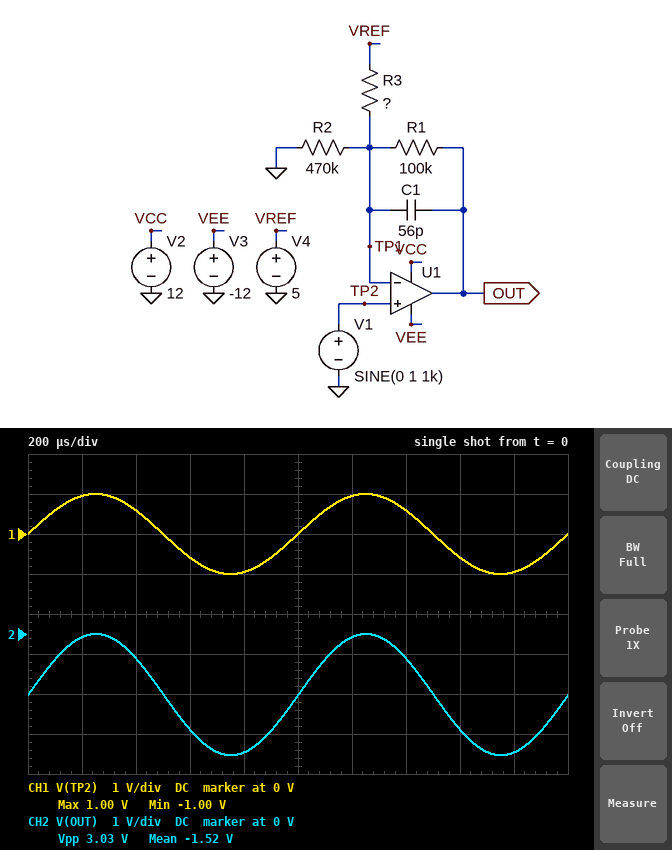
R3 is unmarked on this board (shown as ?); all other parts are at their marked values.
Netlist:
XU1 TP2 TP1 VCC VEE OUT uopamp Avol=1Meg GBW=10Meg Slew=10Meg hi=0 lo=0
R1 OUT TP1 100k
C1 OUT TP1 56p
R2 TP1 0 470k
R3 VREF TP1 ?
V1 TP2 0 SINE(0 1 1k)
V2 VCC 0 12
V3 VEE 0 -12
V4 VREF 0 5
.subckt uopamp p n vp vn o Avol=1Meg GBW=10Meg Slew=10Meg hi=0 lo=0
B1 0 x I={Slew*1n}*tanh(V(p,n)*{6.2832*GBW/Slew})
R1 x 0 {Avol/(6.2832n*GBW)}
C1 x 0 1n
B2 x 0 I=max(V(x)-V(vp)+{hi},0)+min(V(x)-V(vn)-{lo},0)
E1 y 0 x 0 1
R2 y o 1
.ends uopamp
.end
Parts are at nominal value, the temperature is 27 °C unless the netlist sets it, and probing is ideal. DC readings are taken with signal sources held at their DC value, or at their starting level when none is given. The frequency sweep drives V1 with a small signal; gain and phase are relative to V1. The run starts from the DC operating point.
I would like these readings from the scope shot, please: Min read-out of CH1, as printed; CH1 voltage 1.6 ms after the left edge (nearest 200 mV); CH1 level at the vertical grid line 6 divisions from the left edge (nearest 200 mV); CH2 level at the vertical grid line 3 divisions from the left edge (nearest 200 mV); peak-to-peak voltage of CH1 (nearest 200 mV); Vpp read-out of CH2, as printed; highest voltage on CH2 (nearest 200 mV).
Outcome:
-1.00 V
-600 mV
1.0 V
-2.4 V
2.0 V
3.03 V
0 V
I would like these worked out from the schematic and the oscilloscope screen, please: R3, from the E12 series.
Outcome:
330 kΩ
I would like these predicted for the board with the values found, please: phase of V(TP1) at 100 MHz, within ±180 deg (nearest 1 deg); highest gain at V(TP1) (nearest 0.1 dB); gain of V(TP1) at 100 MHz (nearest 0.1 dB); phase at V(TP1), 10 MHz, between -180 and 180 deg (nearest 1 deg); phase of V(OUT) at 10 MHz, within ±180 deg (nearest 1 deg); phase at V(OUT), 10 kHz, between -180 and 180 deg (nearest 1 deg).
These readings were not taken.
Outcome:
-84 deg
0 dB
-20.0 dB
-45 deg
-45 deg
-6 deg
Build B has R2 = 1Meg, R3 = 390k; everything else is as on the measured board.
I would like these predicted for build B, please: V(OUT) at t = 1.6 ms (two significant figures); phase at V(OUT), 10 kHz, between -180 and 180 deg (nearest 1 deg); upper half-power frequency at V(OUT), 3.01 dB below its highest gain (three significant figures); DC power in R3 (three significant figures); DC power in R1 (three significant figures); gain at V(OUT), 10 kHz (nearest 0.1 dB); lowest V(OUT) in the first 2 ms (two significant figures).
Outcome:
-2.1 V
-5 deg
2.92 MHz
64.1 µW
16.4 µW
2.4 dB
-2.6 V
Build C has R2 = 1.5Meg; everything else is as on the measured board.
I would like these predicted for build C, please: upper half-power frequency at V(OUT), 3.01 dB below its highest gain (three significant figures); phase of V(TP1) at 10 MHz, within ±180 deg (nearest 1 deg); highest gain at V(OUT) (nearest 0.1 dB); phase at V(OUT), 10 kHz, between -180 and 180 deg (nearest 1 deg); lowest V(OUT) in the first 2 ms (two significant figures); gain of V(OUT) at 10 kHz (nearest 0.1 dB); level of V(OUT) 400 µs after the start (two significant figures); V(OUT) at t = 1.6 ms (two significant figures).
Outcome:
2.53 MHz
-45 deg
2.7 dB
-5 deg
-2.9 V
2.5 dB
-700 mV
-2.3 V
